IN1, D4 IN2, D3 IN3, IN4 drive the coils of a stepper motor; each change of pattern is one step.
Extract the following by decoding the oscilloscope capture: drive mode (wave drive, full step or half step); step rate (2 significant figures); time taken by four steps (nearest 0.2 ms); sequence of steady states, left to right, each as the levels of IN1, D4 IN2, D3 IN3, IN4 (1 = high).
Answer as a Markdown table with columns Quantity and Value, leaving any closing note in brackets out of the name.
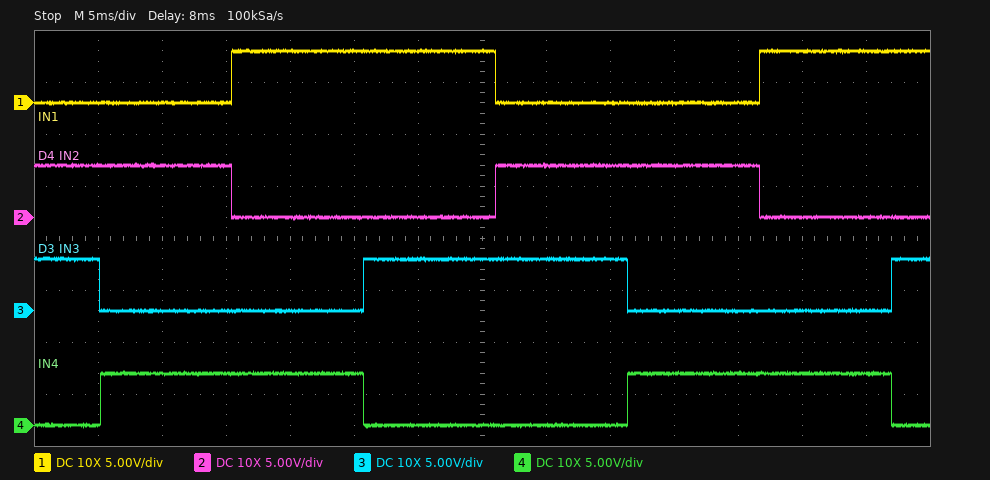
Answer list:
| Quantity | Value |
|---|---|
| drive mode | full step |
| step rate | 97 steps/s |
| time taken by four steps | 41.2 ms |
| sequence of steady states, left to right, each as the levels of IN1, D4 IN2, D3 IN3, IN4 | 0110 0101 1001 1010 0110 0101 1001 1010 |
